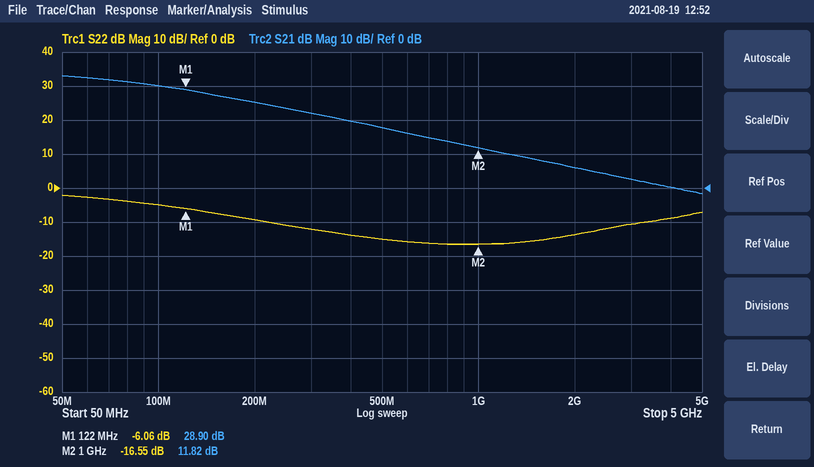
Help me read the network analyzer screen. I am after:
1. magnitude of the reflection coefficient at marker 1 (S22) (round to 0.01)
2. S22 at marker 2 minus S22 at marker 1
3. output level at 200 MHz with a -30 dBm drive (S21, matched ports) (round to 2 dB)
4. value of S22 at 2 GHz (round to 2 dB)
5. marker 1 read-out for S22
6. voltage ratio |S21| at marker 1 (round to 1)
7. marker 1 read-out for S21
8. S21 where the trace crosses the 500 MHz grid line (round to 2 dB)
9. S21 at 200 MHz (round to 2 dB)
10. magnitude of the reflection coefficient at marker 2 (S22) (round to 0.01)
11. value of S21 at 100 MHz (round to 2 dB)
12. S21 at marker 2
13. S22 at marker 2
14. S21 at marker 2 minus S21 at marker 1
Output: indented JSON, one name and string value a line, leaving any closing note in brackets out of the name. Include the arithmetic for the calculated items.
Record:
{
  "magnitude of the reflection coefficient at marker 1 (S22)": "10^(-6.06/20) ≈ 0.50",
  "S22 at marker 2 minus S22 at marker 1": "-16.55 − (-6.06) = -10.49 dB",
  "output level at 200 MHz with a -30 dBm drive (S21, matched ports)": "-30 dBm + (26 dB) = -4 dBm",
  "value of S22 at 2 GHz": "-14 dB",
  "marker 1 read-out for S22": "-6.06 dB",
  "voltage ratio |S21| at marker 1": "10^(28.9/20) ≈ 28",
  "marker 1 read-out for S21": "28.90 dB",
  "S21 where the trace crosses the 500 MHz grid line": "18 dB",
  "S21 at 200 MHz": "26 dB",
  "magnitude of the reflection coefficient at marker 2 (S22)": "10^(-16.55/20) ≈ 0.15",
  "value of S21 at 100 MHz": "30 dB",
  "S21 at marker 2": "11.82 dB",
  "S22 at marker 2": "-16.55 dB",
  "S21 at marker 2 minus S21 at marker 1": "11.82 − (28.9) = -17.08 dB"
}
